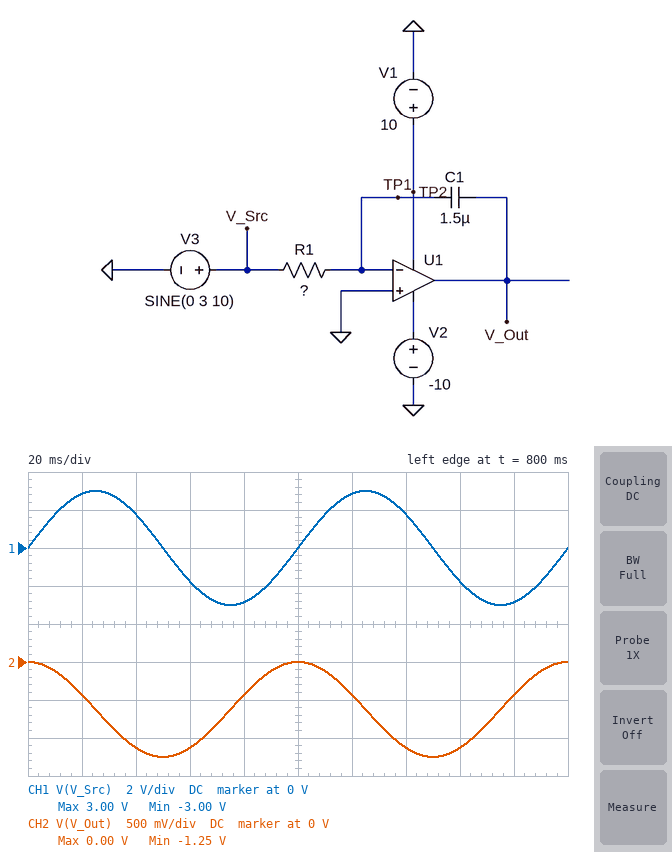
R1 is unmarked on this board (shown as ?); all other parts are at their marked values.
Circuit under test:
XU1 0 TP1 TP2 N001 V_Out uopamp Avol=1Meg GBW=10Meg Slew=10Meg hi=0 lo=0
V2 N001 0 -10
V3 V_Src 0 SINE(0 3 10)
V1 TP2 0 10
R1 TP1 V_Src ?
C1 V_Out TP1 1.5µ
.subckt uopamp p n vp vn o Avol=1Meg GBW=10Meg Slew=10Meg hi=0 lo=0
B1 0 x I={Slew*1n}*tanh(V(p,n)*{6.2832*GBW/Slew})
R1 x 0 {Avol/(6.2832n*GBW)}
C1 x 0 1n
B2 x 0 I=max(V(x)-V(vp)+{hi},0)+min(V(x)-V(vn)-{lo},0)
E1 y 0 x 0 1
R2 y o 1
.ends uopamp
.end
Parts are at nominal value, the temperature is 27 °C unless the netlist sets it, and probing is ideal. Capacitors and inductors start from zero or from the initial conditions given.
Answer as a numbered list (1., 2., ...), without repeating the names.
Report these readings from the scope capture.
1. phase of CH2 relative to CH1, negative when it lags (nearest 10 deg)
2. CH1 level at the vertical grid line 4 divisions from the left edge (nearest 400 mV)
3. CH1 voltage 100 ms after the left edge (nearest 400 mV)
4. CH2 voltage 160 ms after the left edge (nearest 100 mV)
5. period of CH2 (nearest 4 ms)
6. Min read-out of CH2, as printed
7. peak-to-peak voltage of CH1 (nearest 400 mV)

1. 90 deg
2. -2.8 V
3. 0 V
4. -1.1 V
5. 100 ms
6. -1.25 V
7. 6.0 V
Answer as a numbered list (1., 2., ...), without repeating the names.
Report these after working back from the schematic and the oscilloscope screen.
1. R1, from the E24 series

1. 51 kΩ
